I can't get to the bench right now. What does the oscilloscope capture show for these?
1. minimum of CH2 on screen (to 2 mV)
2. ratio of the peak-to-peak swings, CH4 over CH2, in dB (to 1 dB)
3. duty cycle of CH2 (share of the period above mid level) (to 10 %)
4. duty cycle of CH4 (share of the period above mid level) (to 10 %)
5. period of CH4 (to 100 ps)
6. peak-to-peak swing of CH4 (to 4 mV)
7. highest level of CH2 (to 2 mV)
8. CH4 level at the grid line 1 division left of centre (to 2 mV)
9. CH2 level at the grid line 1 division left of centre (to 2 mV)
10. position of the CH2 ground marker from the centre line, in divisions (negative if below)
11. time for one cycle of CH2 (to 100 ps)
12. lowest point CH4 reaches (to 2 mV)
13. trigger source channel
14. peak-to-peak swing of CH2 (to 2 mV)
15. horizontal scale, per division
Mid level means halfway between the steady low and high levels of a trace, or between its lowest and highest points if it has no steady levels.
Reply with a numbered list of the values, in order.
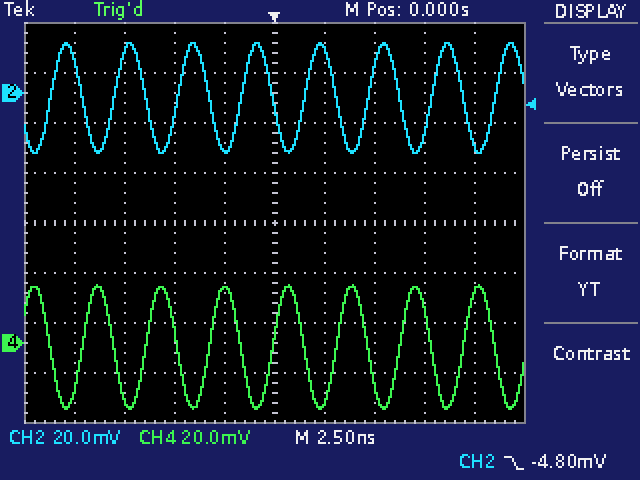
1. -24 mV
2. 1 dB
3. 50 %
4. 50 %
5. 3.2 ns
6. 48 mV
7. 20 mV
8. 22 mV
9. -22 mV
10. +2.6 div
11. 3.2 ns
12. -26 mV
13. CH2
14. 44 mV
15. 2.5 ns
